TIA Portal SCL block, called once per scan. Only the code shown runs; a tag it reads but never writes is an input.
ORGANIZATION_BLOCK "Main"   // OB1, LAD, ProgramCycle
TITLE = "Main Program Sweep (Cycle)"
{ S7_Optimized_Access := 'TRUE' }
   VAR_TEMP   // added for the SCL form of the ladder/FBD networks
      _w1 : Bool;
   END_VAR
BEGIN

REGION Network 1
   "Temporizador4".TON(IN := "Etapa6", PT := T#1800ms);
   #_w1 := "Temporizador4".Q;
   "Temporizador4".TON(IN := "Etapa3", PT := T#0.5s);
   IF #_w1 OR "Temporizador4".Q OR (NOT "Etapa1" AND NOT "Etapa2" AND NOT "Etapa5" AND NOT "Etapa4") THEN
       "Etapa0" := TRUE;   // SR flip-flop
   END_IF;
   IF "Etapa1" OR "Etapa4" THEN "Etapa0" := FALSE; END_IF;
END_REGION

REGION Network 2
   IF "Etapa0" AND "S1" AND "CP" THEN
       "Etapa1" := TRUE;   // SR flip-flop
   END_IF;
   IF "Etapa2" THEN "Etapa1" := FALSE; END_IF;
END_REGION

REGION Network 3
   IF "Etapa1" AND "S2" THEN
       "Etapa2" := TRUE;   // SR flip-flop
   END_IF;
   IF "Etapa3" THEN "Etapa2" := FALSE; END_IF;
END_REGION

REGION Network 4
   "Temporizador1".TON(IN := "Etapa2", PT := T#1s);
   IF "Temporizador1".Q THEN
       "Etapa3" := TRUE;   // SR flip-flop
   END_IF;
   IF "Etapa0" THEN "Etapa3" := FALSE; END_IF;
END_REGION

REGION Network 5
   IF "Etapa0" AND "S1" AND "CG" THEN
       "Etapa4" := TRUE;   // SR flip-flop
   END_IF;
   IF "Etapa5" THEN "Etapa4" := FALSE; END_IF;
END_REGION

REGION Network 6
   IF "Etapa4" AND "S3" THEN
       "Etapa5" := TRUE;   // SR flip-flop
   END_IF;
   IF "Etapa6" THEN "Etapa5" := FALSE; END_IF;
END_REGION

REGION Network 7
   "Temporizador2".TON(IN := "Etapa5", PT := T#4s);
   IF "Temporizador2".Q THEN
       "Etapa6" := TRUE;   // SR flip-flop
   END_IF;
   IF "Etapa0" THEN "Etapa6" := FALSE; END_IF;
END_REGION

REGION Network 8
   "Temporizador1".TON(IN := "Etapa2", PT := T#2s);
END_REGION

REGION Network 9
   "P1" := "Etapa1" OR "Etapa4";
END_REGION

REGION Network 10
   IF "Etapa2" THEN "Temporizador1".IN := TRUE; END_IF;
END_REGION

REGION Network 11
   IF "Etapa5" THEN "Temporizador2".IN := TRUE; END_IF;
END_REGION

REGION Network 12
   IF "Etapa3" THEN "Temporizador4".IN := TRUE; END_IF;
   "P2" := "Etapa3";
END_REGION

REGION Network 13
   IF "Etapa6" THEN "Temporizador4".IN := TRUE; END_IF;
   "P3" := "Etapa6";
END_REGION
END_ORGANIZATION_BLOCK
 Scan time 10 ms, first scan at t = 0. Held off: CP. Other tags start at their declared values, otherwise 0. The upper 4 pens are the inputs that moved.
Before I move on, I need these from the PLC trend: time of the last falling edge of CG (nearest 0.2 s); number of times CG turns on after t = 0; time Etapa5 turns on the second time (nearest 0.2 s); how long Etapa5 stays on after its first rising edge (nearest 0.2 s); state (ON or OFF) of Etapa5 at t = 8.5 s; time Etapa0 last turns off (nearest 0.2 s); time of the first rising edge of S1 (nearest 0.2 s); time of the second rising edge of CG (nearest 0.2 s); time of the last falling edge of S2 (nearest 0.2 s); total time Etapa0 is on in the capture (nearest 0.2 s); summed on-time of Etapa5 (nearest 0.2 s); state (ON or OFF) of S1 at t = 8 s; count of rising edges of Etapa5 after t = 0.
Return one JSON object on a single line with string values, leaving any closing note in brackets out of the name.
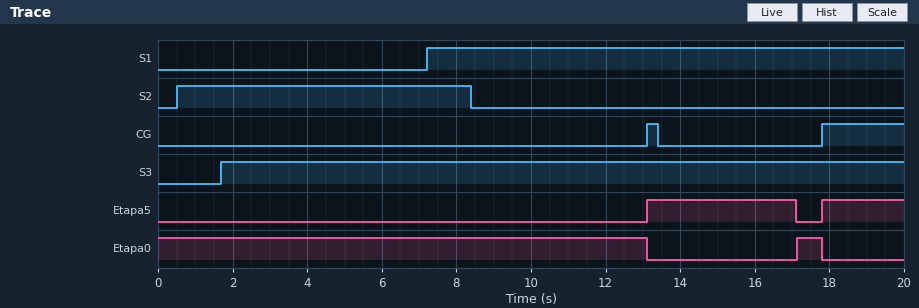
{"time of the last falling edge of CG": "13.4 s", "number of times CG turns on after t = 0": "2", "time Etapa5 turns on the second time": "17.8 s", "how long Etapa5 stays on after its first rising edge": "4.0 s", "state (ON or OFF) of Etapa5 at t = 8.5 s": "OFF", "time Etapa0 last turns off": "17.8 s", "time of the first rising edge of S1": "7.2 s", "time of the second rising edge of CG": "17.8 s", "time of the last falling edge of S2": "8.4 s", "total time Etapa0 is on in the capture": "13.8 s", "summed on-time of Etapa5": "6.2 s", "state (ON or OFF) of S1 at t = 8 s": "ON", "count of rising edges of Etapa5 after t = 0": "2"}
